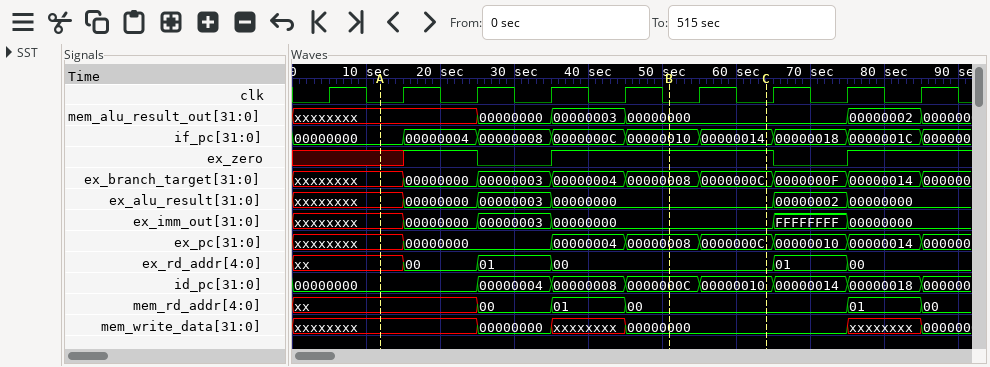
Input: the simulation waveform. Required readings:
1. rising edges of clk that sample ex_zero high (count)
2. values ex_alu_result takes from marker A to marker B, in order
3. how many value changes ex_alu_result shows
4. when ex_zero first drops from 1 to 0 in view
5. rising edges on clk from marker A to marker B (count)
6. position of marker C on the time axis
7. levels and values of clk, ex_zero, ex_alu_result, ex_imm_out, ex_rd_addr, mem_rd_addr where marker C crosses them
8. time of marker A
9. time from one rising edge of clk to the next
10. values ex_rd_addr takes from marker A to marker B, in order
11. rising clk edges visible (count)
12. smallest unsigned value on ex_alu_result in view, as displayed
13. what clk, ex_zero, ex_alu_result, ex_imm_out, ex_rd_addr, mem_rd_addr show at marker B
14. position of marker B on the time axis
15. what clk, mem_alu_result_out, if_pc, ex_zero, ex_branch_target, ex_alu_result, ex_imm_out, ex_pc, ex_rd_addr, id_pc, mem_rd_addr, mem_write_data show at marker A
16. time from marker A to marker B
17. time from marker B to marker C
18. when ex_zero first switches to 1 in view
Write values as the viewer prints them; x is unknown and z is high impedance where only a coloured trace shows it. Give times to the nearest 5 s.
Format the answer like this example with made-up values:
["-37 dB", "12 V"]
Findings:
["5", "xxxxxxxx, 00000000, 00000003, 00000000", "5", "25 s", "4", "65 s", "clk=0, ex_zero=1, ex_alu_result=00000000, ex_imm_out=00000000, ex_rd_addr=00, mem_rd_addr=00", "10 s", "10 s", "xx, 00, 01, 00", "9", "00000000", "clk=0, ex_zero=1, ex_alu_result=00000000, ex_imm_out=00000000, ex_rd_addr=00, mem_rd_addr=00", "50 s", "clk=0, mem_alu_result_out=xxxxxxxx, if_pc=00000000, ex_zero=x, ex_branch_target=xxxxxxxx, ex_alu_result=xxxxxxxx, ex_imm_out=xxxxxxxx, ex_pc=xxxxxxxx, ex_rd_addr=xx, id_pc=00000000, mem_rd_addr=xx, mem_write_data=xxxxxxxx", "40 s", "15 s", "15 s"]
